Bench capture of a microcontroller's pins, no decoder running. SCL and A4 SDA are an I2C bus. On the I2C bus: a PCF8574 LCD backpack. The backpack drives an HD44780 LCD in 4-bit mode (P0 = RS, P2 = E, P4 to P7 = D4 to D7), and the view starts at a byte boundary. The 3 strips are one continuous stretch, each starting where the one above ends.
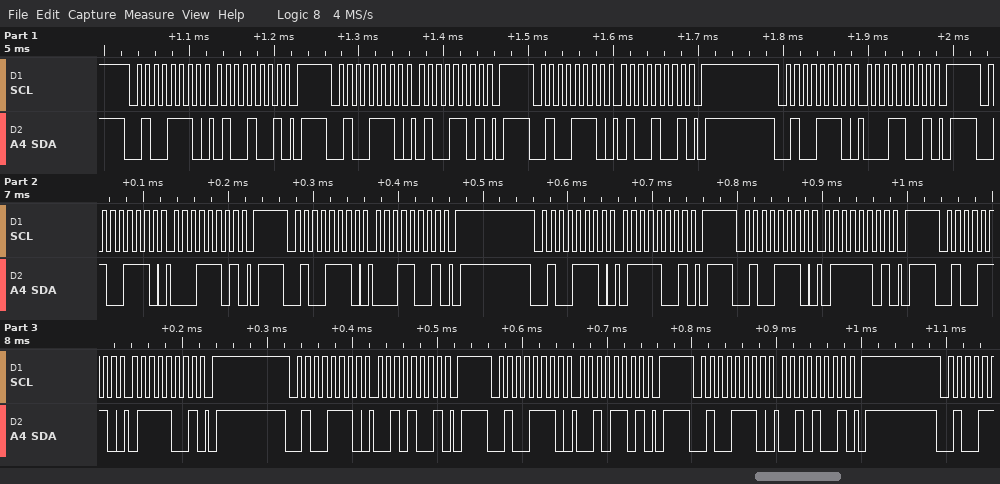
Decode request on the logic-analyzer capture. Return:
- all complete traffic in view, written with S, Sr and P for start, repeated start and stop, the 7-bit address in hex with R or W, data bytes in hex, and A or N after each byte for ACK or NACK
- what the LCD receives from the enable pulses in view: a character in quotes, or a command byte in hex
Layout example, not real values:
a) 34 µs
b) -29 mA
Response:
a) S 27W A 49 A P S 27W A 4D A P S 27W A 49 A P S 27W A 19 A P S 27W A 1D A P S 27W A 19 A P S 27W A 79 A P S 27W A 7D A P S 27W A 79 A P S 27W A 29 A P S 27W A 2D A P S 27W A 29 A P
b) 'A' 'r'
